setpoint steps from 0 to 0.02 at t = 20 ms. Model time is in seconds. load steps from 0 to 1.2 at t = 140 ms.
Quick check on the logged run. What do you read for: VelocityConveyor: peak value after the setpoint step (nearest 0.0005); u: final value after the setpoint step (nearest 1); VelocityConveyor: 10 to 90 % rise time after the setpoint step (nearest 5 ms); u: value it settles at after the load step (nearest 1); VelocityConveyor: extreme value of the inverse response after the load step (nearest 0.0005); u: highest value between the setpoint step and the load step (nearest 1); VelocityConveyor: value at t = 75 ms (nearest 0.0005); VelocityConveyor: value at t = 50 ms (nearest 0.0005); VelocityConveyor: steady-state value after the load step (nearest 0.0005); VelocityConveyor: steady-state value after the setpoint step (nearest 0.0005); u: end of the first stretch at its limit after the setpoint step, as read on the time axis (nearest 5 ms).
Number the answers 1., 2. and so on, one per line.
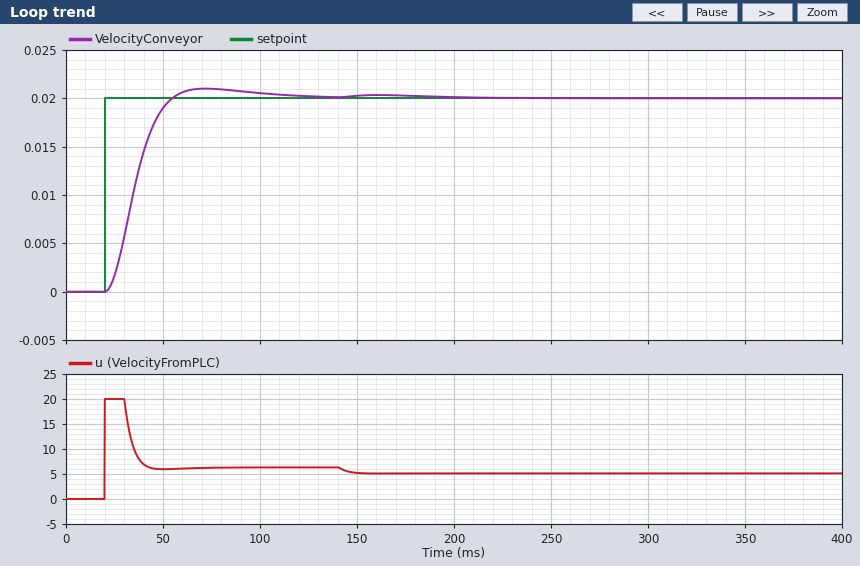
1. 0.0210
2. 6
3. 20 ms
4. 5
5. 0.0205
6. 20
7. 0.0210
8. 0.0190
9. 0.0200
10. 0.0200
11. 30 ms
